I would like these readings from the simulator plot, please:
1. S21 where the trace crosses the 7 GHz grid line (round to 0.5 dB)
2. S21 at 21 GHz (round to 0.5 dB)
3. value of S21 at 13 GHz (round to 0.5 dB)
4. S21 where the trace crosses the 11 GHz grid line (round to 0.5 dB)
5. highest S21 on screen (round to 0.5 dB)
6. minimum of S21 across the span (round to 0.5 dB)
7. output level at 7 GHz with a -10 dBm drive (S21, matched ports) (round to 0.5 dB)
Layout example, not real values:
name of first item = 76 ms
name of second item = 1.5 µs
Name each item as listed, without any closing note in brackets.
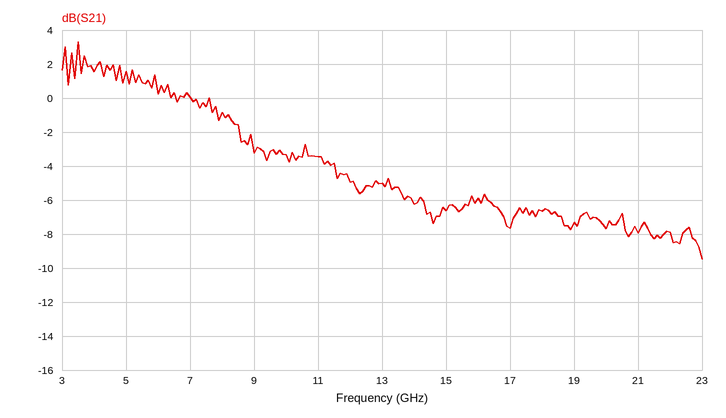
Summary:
S21 where the trace crosses the 7 GHz grid line = 0.0 dB
S21 at 21 GHz = -8.0 dB
value of S21 at 13 GHz = -5.0 dB
S21 where the trace crosses the 11 GHz grid line = -3.5 dB
highest S21 on screen = 3.5 dB
minimum of S21 across the span = -9.5 dB
output level at 7 GHz with a -10 dBm drive (S21, matched ports) = -10.0 dBm
